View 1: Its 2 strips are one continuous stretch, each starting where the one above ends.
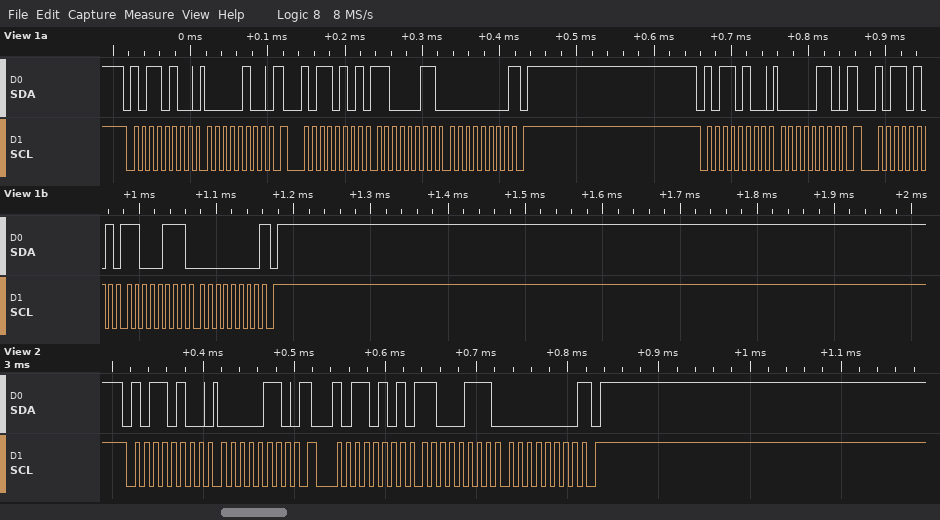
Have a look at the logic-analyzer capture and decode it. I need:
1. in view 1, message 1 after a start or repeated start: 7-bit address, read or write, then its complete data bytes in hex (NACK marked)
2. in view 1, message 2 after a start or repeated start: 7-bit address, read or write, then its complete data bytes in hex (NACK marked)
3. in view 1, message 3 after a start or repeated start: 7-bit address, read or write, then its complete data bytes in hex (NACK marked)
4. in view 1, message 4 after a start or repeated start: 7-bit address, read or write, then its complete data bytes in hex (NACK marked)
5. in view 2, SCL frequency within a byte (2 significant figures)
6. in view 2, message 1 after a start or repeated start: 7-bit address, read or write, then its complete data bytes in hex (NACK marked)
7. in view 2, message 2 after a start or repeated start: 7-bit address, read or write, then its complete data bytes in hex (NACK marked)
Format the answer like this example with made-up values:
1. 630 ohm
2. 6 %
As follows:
1. 0x5A write: 04
2. 0x5A read: C3 00 NACK
3. 0x5A write: 06
4. 0x5A read: C7 00 NACK
5. 100 kHz
6. 0x5A write: 06
7. 0x5A read: C7 00 NACK
